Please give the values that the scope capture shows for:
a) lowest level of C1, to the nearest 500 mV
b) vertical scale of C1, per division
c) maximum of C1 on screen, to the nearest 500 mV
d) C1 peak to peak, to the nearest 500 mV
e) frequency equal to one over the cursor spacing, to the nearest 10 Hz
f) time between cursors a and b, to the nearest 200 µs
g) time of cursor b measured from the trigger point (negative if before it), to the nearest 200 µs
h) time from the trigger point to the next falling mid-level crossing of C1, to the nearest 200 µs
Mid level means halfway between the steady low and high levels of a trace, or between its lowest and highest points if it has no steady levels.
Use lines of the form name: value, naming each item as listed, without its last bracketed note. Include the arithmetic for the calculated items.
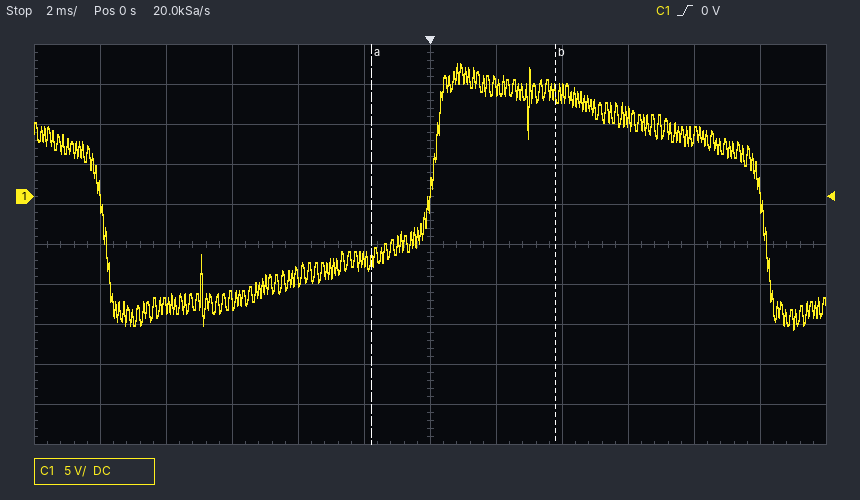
lowest level of C1, to the nearest 500 mV: -16.5 V
vertical scale of C1, per division: 5 V
maximum of C1 on screen, to the nearest 500 mV: 16.5 V
C1 peak to peak, to the nearest 500 mV: 16.5 V − (-16.5 V) = 33.0 V
frequency equal to one over the cursor spacing, to the nearest 10 Hz: 1 / 5.6 ms ≈ 180 Hz
time between cursors a and b, to the nearest 200 µs: 5.6 ms
time of cursor b measured from the trigger point (negative if before it), to the nearest 200 µs: +3.8 ms
time from the trigger point to the next falling mid-level crossing of C1, to the nearest 200 µs: 10.0 ms
